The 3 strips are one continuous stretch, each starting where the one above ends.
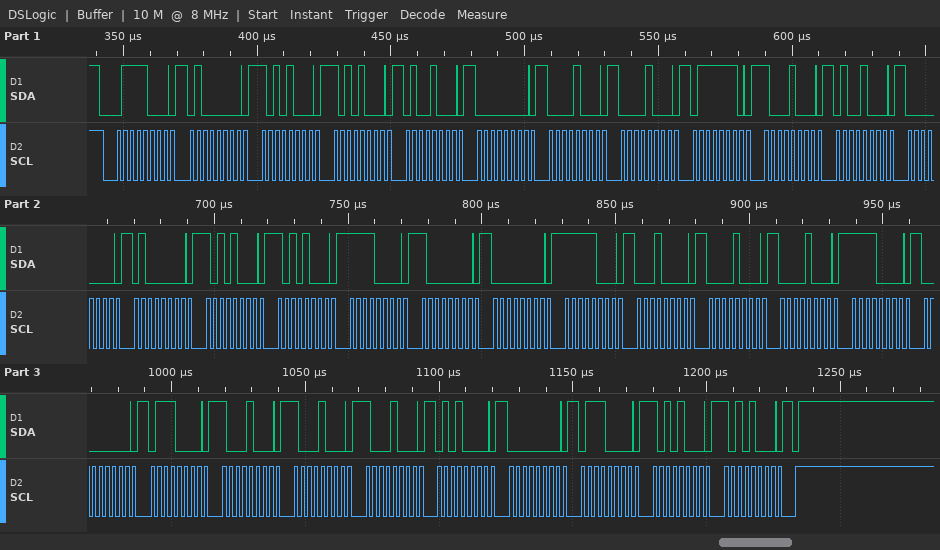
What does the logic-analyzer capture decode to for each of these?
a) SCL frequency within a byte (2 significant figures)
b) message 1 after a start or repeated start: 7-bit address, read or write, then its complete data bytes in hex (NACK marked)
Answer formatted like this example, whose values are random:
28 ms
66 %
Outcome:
400 kHz
0x3C write: 40 A8 A8 48 00 08 08 7E 88 48 00 40 A8 A8 F0 80 00 F8 10 08 08 F0 00 70 88 88 88 50 00 70 A8 A8
